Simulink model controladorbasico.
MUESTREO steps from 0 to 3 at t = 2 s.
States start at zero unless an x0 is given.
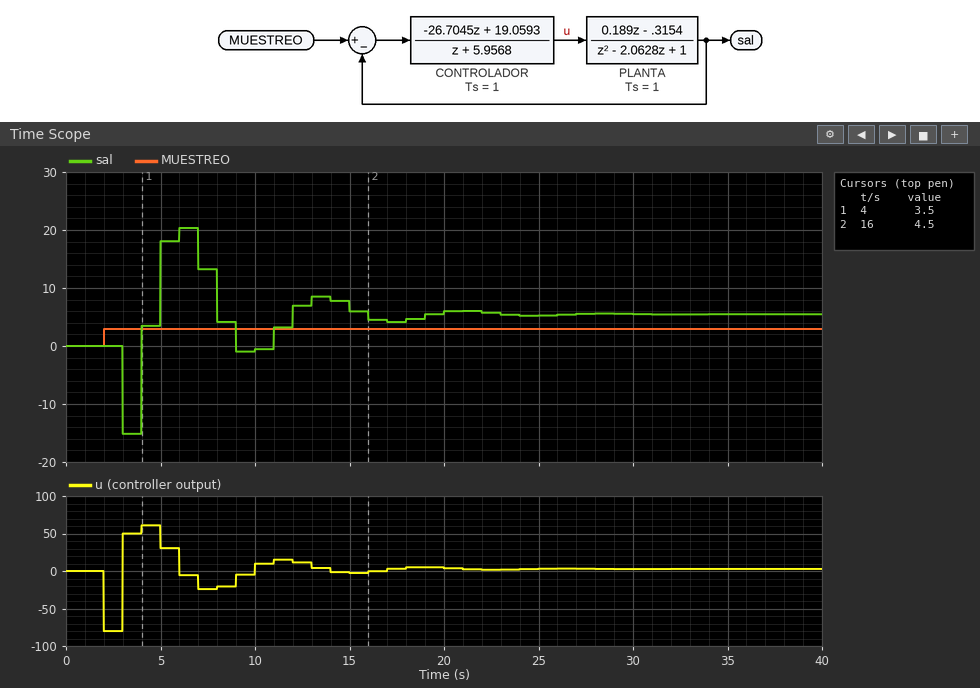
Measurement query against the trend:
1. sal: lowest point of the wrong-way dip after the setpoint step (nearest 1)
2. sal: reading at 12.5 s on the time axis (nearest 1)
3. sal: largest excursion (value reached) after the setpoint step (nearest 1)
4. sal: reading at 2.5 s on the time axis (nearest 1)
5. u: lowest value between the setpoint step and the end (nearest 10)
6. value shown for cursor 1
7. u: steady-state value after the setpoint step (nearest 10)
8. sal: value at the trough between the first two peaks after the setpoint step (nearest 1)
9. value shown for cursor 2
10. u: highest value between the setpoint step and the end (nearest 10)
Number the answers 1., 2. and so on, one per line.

1. -15
2. 7
3. 20
4. 0
5. -80
6. 3.5
7. 0
8. -1
9. 4.5
10. 60
